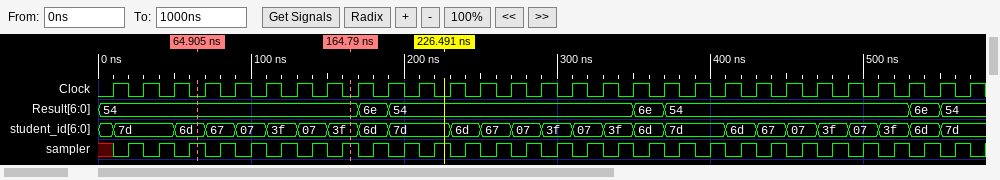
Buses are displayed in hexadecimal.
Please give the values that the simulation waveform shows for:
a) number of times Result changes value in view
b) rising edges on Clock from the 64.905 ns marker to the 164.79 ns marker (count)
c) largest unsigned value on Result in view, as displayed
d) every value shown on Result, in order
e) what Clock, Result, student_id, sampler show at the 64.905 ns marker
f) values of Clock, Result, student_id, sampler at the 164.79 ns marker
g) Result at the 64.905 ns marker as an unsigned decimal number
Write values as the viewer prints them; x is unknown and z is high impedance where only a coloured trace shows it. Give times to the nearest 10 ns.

6
5
6e
54, 6e, 54, 6e, 54, 6e, 54
Clock=0, Result=54, student_id=6d, sampler=1
Clock=0, Result=54, student_id=3f, sampler=1
84
